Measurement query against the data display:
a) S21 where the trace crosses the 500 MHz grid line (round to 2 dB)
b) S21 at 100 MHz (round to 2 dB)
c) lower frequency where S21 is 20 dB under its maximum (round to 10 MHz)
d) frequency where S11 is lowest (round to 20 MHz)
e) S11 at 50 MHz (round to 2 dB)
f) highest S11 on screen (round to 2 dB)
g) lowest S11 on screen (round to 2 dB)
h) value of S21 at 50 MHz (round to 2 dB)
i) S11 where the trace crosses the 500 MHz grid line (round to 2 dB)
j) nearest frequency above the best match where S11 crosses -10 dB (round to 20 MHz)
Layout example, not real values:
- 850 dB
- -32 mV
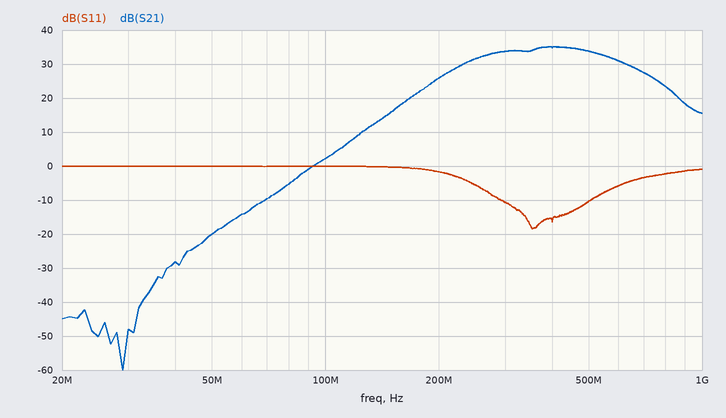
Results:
- 34 dB
- 2 dB
- 150 MHz
- 360 MHz
- 0 dB
- 0 dB
- -18 dB
- -20 dB
- -10 dB
- 500 MHz
